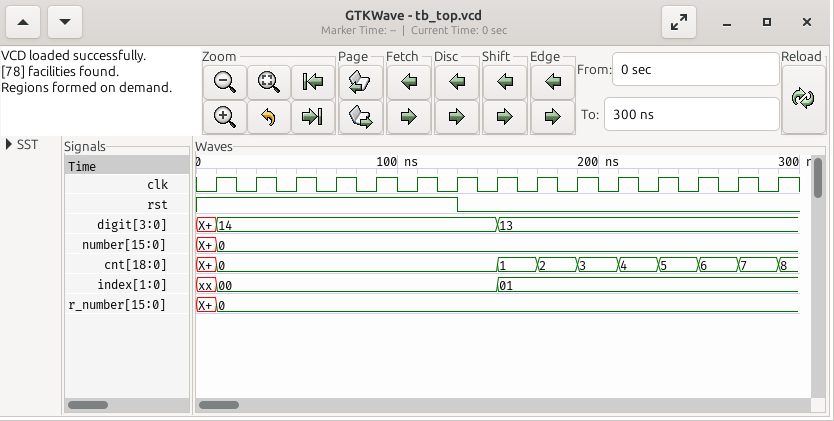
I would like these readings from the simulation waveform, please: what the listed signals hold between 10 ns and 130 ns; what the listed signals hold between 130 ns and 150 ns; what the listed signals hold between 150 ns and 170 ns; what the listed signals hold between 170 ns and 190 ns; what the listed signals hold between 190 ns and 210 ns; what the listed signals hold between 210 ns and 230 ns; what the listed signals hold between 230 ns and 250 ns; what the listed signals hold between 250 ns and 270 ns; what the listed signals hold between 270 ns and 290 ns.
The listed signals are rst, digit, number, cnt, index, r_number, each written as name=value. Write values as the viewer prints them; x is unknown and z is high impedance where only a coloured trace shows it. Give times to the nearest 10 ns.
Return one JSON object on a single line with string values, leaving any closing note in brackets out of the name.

{"what the listed signals hold between 10 ns and 130 ns": "rst=1, digit=14, number=0, cnt=0, index=00, r_number=0", "what the listed signals hold between 130 ns and 150 ns": "rst=0, digit=14, number=0, cnt=0, index=00, r_number=0", "what the listed signals hold between 150 ns and 170 ns": "rst=0, digit=13, number=0, cnt=1, index=01, r_number=0", "what the listed signals hold between 170 ns and 190 ns": "rst=0, digit=13, number=0, cnt=2, index=01, r_number=0", "what the listed signals hold between 190 ns and 210 ns": "rst=0, digit=13, number=0, cnt=3, index=01, r_number=0", "what the listed signals hold between 210 ns and 230 ns": "rst=0, digit=13, number=0, cnt=4, index=01, r_number=0", "what the listed signals hold between 230 ns and 250 ns": "rst=0, digit=13, number=0, cnt=5, index=01, r_number=0", "what the listed signals hold between 250 ns and 270 ns": "rst=0, digit=13, number=0, cnt=6, index=01, r_number=0", "what the listed signals hold between 270 ns and 290 ns": "rst=0, digit=13, number=0, cnt=7, index=01, r_number=0"}
